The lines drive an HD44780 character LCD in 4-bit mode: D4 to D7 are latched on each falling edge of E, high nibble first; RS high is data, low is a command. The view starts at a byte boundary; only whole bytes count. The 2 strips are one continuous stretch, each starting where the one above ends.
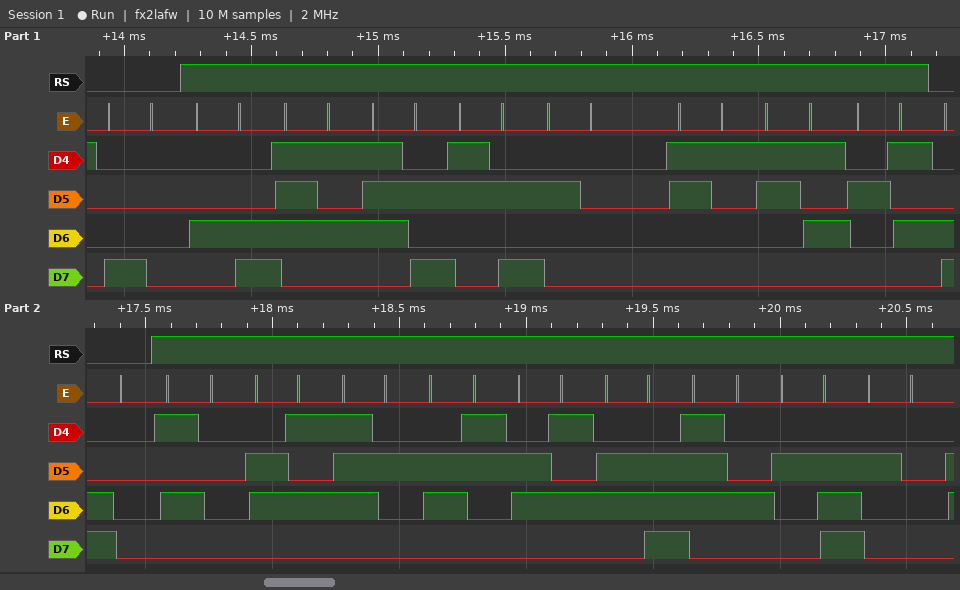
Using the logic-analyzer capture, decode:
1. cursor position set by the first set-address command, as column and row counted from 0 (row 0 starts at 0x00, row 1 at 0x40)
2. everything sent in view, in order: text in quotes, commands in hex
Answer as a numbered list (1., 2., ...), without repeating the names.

1. column 0, row 0
2. 0x80 "Luz: 15%" 0xC0 "Percent. "
